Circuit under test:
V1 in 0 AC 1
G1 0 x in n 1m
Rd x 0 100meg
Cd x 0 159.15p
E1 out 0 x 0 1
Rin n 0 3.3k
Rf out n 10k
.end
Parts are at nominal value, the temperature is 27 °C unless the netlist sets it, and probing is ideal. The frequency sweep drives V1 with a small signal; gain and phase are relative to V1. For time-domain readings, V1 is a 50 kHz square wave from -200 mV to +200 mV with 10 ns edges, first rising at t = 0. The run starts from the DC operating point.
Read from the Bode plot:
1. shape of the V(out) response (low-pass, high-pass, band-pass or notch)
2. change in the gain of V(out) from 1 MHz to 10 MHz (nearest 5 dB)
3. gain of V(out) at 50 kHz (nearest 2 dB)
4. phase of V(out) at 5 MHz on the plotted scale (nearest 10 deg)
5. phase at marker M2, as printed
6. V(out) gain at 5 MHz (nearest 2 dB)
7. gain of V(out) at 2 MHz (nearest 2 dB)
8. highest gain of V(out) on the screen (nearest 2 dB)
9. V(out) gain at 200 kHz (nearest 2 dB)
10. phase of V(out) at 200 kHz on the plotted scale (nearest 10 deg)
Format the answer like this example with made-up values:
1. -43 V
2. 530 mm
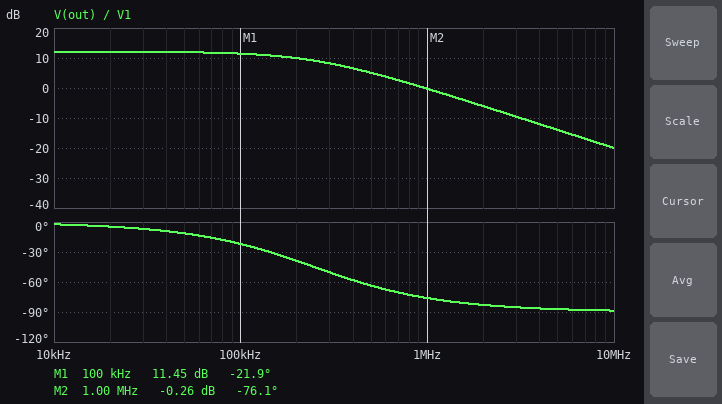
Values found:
1. low-pass
2. -20 dB
3. 12 dB
4. -90 deg
5. -76.1 deg
6. -14 dB
7. -6 dB
8. 12 dB
9. 10 dB
10. -40 deg
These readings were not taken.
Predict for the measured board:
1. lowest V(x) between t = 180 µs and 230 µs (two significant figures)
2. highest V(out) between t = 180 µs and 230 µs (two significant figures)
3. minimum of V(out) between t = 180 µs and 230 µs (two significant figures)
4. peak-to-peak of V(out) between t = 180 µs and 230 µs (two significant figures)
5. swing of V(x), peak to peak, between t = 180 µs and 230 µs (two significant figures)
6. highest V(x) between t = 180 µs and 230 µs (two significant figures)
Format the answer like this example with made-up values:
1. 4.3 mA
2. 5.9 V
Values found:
1. -810 mV
2. 810 mV
3. -810 mV
4. 1.6 V
5. 1.6 V
6. 810 mV
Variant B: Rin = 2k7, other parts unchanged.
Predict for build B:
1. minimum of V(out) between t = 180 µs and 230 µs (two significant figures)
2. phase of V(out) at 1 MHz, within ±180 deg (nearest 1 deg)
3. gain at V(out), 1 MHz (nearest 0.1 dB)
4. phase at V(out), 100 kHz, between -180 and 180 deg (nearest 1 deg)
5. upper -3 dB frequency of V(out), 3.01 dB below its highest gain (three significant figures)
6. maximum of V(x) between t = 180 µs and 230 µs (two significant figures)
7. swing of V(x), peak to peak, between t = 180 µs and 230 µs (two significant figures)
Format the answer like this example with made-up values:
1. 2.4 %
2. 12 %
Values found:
1. -940 mV
2. -78 deg
3. -0.2 dB
4. -25 deg
5. 213 kHz
6. 940 mV
7. 1.9 V
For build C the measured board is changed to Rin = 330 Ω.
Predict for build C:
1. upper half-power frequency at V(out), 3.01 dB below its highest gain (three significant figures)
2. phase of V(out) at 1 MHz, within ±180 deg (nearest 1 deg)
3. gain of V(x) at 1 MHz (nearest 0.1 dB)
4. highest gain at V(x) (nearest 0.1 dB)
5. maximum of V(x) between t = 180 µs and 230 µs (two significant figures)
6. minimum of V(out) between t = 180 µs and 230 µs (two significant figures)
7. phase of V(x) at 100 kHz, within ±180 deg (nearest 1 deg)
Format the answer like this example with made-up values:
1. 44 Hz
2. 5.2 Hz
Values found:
1. 32.0 kHz
2. -88 deg
3. 0 dB
4. 29.9 dB
5. 4.8 V
6. -4.8 V
7. -72 deg
